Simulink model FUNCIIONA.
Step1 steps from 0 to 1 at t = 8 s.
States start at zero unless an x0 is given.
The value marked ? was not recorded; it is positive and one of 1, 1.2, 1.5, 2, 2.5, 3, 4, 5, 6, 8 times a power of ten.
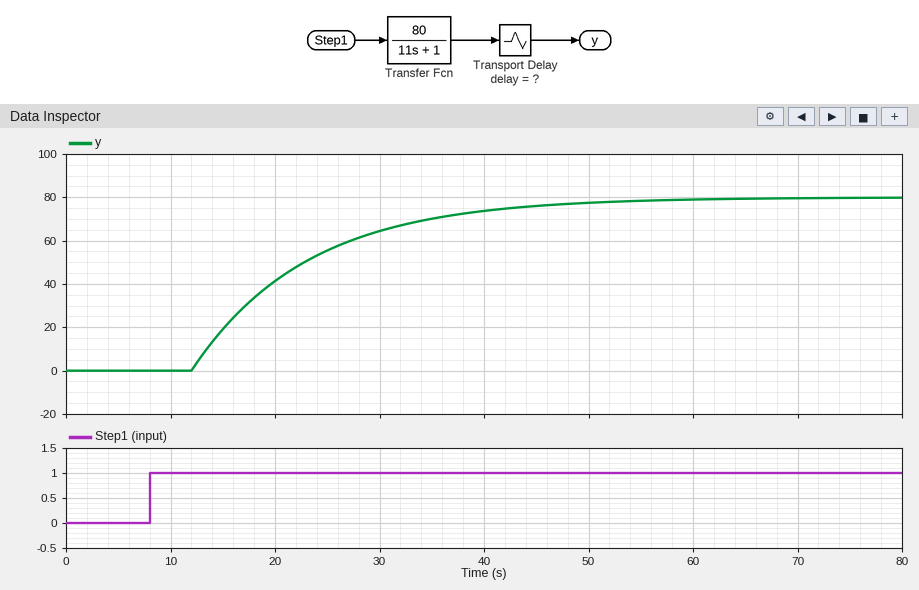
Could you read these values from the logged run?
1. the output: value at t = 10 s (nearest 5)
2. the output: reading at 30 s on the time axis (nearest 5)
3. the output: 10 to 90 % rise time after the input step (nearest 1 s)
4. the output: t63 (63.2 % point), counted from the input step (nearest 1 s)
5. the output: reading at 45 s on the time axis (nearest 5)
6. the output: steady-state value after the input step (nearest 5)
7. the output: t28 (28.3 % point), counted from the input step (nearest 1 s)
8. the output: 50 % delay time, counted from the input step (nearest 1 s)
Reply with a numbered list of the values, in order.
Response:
1. 0
2. 65
3. 24 s
4. 15 s
5. 75
6. 80
7. 8 s
8. 12 s
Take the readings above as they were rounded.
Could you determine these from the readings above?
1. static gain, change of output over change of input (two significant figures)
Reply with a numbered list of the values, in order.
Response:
1. 80
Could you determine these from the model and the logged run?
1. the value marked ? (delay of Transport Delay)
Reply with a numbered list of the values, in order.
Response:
1. 4
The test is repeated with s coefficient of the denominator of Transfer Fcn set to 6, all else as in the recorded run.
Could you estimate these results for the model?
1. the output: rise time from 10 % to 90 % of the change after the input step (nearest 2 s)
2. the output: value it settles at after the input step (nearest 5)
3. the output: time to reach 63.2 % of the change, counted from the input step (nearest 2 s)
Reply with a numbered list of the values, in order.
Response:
1. 14 s
2. 80
3. 10 s
